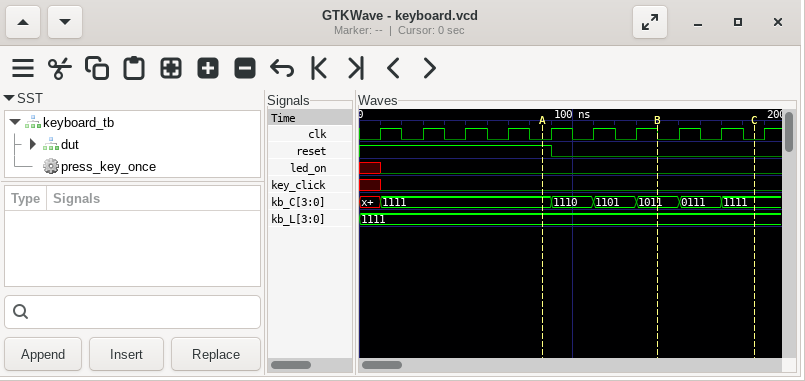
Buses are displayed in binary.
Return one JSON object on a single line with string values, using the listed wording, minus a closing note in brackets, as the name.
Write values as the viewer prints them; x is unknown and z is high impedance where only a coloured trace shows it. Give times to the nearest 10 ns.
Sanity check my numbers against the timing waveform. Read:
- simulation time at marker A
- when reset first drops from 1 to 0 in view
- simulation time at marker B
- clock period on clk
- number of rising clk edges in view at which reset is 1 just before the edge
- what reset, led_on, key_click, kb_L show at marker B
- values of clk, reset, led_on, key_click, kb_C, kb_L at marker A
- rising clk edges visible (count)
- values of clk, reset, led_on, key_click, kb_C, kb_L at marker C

{"simulation time at marker A": "90 ns", "when reset first drops from 1 to 0 in view": "90 ns", "simulation time at marker B": "140 ns", "clock period on clk": "20 ns", "number of rising clk edges in view at which reset is 1 just before the edge": "5", "what reset, led_on, key_click, kb_L show at marker B": "reset=0, led_on=0, key_click=0, kb_L=1111", "values of clk, reset, led_on, key_click, kb_C, kb_L at marker A": "clk=0, reset=1, led_on=0, key_click=0, kb_C=1111, kb_L=1111", "rising clk edges visible": "10", "values of clk, reset, led_on, key_click, kb_C, kb_L at marker C": "clk=0, reset=0, led_on=0, key_click=0, kb_C=1111, kb_L=1111"}
